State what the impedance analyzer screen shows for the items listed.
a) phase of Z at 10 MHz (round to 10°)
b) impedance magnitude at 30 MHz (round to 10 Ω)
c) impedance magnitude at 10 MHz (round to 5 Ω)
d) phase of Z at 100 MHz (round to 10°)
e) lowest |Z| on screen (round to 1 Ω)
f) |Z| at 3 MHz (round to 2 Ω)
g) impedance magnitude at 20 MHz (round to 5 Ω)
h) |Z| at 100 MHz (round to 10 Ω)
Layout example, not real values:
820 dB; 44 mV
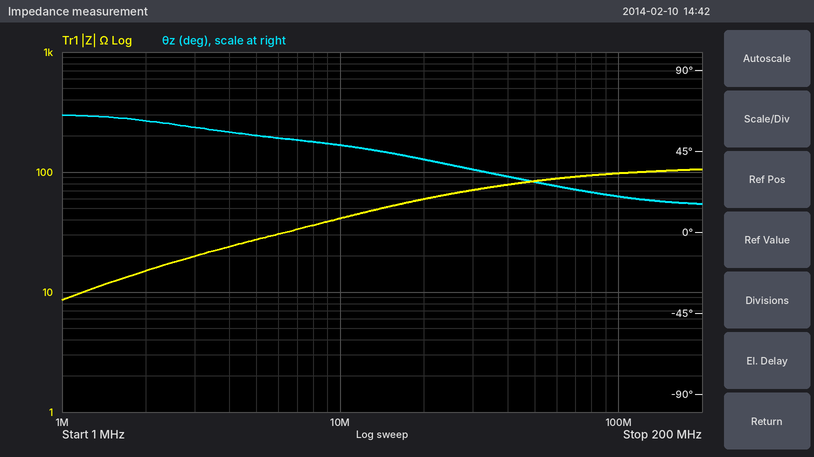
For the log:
50°; 70 Ω; 40 Ω; 20°; 9 Ω; 20 Ω; 60 Ω; 100 Ω
